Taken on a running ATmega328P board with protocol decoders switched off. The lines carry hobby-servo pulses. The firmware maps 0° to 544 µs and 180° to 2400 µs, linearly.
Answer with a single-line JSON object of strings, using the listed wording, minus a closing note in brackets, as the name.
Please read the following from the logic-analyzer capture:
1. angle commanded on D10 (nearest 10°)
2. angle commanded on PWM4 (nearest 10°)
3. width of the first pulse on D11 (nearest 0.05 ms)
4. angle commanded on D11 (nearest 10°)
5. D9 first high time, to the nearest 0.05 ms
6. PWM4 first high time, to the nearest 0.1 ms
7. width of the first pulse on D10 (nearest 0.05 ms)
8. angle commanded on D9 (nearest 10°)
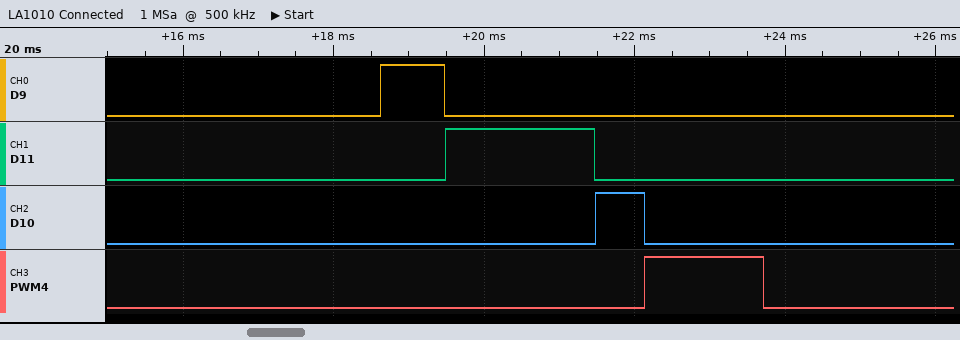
{"angle commanded on D10": "10°", "angle commanded on PWM4": "100°", "width of the first pulse on D11": "2.00 ms", "angle commanded on D11": "140°", "D9 first high time, to the nearest 0.05 ms": "0.85 ms", "PWM4 first high time, to the nearest 0.1 ms": "1.6 ms", "width of the first pulse on D10": "0.65 ms", "angle commanded on D9": "30°"}
